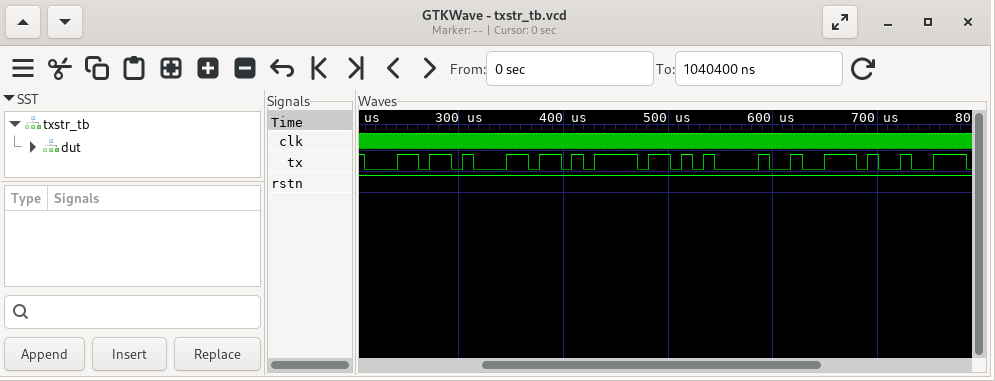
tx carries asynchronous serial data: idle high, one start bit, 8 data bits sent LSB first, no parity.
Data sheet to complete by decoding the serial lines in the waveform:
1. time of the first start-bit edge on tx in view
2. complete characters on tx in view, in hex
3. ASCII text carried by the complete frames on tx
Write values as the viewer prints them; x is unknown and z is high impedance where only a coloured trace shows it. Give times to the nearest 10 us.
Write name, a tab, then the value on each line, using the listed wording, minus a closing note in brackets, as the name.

time of the first start-bit edge on tx in view	210 us
complete characters on tx in view, in hex	6C, 6C, 6F, 21, 2E
ASCII text carried by the complete frames on tx	"llo!."
